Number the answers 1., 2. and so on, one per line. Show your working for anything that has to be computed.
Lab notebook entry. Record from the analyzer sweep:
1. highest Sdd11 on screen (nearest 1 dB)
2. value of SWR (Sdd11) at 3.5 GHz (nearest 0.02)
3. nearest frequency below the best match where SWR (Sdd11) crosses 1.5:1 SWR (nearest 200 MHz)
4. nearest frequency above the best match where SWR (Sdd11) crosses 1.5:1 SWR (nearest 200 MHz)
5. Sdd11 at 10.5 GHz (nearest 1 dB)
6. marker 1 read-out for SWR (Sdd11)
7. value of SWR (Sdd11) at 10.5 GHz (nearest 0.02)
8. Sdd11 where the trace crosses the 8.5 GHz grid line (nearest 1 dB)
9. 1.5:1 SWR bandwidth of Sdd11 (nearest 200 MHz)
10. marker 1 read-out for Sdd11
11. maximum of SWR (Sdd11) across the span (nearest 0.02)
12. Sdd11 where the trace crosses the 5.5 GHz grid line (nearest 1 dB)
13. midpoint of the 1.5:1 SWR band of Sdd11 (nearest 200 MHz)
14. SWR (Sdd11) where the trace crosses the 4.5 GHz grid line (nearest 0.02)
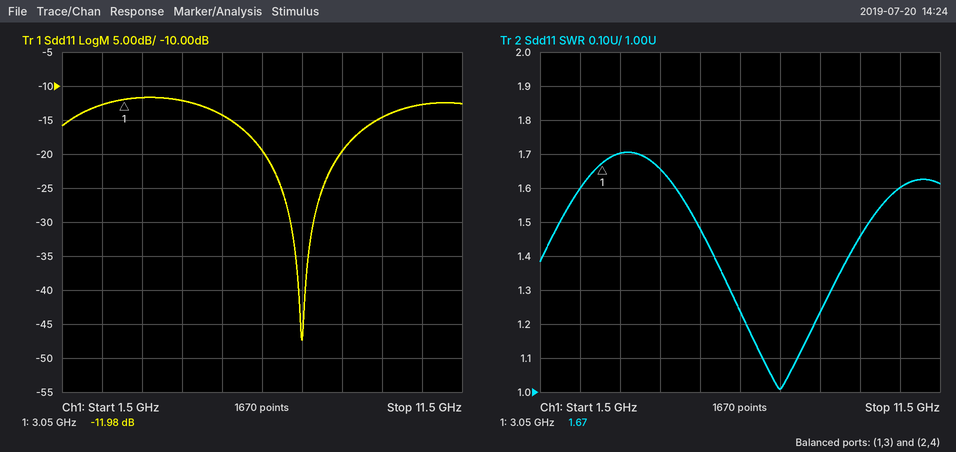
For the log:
1. -12 dB
2. 1.70
3. 5.4 GHz
4. 9.8 GHz
5. -13 dB
6. 1.67
7. 1.60
8. -20 dB
9. 9.8 GHz − 5.4 GHz = 4.4 GHz
10. -11.98 dB
11. 1.70
12. -14 dB
13. 7.6 GHz
14. 1.66
